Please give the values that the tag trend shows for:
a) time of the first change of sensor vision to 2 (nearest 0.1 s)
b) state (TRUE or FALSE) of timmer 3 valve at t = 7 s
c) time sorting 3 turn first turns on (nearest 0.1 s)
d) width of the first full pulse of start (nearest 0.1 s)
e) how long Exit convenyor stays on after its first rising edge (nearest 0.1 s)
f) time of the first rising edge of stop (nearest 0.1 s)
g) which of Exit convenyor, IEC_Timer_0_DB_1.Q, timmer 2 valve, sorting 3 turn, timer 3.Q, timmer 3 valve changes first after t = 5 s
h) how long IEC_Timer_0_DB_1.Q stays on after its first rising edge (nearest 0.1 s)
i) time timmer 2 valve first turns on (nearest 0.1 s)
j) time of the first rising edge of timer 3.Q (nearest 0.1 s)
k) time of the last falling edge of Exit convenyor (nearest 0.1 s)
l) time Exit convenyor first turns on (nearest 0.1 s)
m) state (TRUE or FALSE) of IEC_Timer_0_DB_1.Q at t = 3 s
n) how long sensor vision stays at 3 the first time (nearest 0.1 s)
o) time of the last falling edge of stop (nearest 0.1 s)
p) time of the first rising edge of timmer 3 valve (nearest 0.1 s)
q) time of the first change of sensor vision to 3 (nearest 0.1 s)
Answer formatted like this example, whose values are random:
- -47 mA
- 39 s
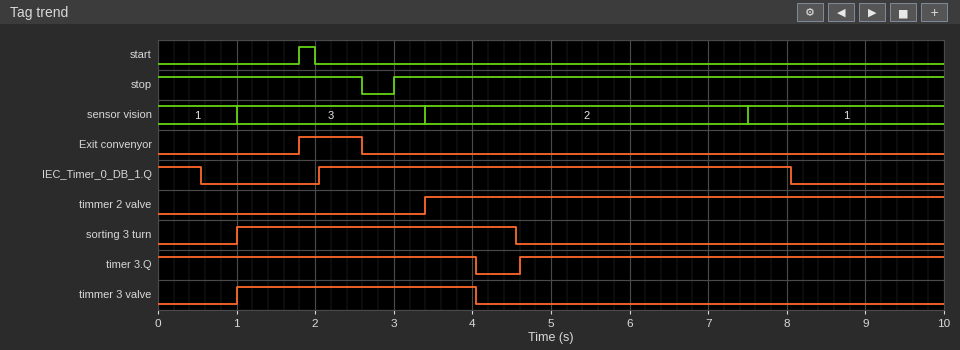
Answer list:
- 3.4 s
- FALSE
- 1.0 s
- 0.2 s
- 0.8 s
- 3.0 s
- IEC_Timer_0_DB_1.Q
- 6.0 s
- 3.4 s
- 4.6 s
- 2.6 s
- 1.8 s
- TRUE
- 2.4 s
- 2.6 s
- 1.0 s
- 1.0 s
